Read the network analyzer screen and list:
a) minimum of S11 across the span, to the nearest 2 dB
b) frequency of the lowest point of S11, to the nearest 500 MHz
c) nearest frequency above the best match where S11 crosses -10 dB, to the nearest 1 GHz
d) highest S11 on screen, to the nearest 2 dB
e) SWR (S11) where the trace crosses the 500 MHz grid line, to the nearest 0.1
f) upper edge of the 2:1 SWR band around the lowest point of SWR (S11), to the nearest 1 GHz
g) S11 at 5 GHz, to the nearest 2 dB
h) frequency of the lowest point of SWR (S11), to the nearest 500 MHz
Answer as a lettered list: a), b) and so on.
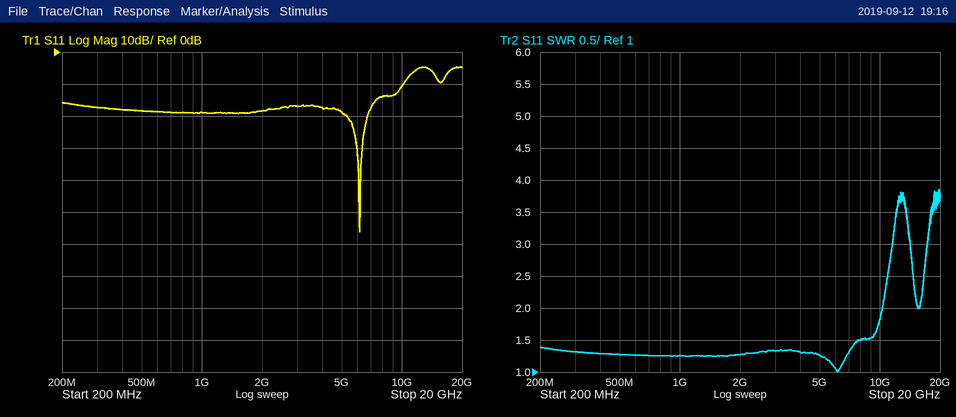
a) -56 dB
b) 6.0 GHz
c) 10 GHz
d) -4 dB
e) 1.3
f) 10 GHz
g) -18 dB
h) 6.0 GHz
